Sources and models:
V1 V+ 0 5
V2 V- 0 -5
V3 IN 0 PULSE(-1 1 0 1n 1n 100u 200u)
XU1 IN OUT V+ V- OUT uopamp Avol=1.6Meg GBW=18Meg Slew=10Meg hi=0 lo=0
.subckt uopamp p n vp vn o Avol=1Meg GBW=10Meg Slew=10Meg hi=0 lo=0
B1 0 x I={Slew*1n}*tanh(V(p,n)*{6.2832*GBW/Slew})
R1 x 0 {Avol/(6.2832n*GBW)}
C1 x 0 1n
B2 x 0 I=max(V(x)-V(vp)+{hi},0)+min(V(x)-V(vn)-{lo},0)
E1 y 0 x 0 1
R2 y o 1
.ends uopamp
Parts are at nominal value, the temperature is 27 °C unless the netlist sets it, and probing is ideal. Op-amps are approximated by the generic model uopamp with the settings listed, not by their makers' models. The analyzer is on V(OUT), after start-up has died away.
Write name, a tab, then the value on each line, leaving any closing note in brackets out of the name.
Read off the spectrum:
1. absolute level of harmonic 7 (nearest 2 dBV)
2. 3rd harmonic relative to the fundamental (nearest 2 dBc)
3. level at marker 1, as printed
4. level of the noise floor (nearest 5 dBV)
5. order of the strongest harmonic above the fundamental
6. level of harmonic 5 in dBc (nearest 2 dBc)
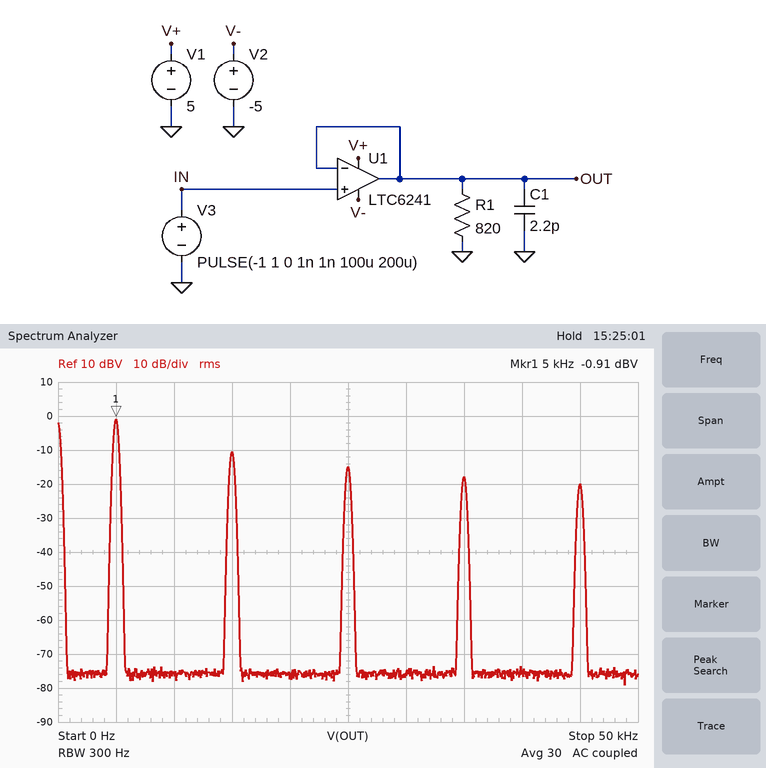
absolute level of harmonic 7	-18 dBV
3rd harmonic relative to the fundamental	-10 dBc
level at marker 1, as printed	-0.91 dBV
level of the noise floor	-75 dBV
order of the strongest harmonic above the fundamental	3
level of harmonic 5 in dBc	-14 dBc
